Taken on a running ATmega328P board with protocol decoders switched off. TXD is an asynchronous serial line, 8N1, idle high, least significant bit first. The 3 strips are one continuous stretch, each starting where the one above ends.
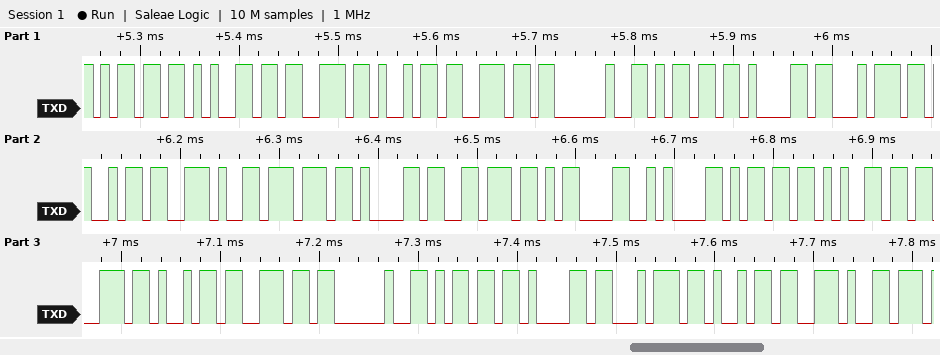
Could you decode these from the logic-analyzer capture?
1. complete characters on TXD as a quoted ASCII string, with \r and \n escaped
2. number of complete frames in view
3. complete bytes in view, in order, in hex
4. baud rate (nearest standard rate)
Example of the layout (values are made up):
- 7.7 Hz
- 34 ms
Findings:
- "mesin mati.wav\r\nmesin mati."
- 27
- 6D 65 73 69 6E 20 6D 61 74 69 2E 77 61 76 0D 0A 6D 65 73 69 6E 20 6D 61 74 69 2E
- 115200 baud
